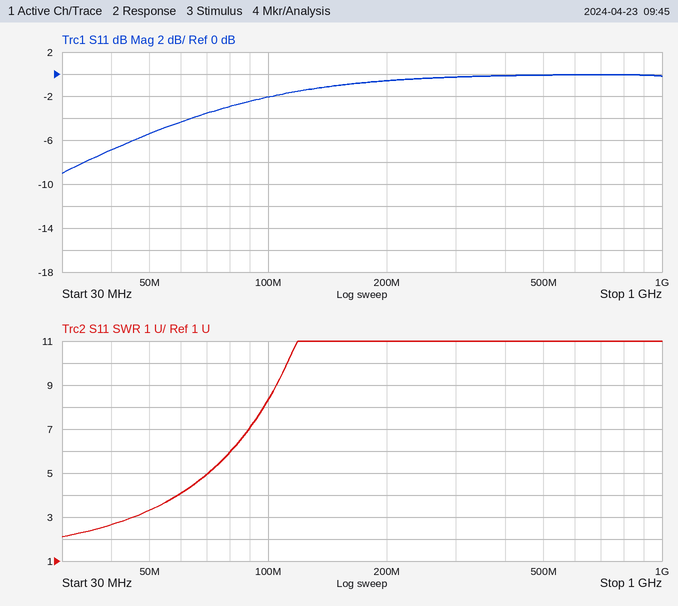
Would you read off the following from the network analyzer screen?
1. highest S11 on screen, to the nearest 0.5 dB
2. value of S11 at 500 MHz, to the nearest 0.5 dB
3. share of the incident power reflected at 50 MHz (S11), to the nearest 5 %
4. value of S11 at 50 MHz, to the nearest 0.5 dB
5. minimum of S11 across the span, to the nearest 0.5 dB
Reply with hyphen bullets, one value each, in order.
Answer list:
- 0.0 dB
- 0.0 dB
- 30 %
- -5.5 dB
- -9.0 dB
